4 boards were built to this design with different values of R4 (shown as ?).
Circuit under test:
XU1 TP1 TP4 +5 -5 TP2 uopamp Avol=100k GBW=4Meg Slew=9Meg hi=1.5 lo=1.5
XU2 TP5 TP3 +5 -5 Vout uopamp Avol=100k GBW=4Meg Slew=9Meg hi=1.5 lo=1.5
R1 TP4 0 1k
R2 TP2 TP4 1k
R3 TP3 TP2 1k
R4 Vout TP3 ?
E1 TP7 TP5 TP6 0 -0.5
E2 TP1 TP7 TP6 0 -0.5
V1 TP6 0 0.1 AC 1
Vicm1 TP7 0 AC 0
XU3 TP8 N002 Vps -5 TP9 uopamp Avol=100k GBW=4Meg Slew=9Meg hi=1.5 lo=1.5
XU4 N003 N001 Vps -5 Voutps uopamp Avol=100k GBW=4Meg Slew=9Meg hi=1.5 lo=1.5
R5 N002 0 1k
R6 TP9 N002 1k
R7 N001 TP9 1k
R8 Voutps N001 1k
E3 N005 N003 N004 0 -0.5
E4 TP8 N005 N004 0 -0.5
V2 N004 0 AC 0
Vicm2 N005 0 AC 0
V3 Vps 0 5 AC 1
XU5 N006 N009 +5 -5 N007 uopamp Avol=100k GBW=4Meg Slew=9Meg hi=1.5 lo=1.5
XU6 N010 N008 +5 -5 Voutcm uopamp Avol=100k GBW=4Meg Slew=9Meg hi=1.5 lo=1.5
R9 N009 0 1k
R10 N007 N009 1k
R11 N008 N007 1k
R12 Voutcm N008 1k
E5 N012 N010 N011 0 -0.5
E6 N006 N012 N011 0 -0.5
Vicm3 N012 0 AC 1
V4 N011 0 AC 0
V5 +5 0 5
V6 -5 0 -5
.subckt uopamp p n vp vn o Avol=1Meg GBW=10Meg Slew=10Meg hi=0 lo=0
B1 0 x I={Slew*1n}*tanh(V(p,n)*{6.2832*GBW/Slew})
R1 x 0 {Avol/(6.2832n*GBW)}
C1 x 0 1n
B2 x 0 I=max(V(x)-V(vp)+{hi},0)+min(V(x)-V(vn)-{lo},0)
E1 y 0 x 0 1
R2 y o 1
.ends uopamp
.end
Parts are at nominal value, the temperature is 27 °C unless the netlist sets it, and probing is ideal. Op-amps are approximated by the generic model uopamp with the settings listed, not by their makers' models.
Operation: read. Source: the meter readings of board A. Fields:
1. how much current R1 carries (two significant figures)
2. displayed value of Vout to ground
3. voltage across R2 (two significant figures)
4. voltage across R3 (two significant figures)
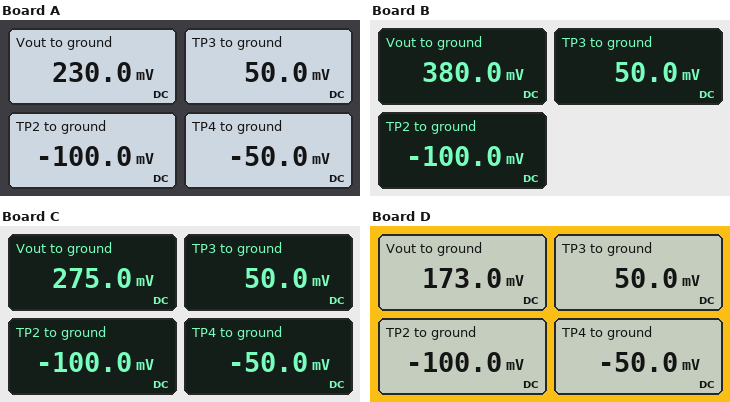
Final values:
50 µA
230.0 mV
50 mV
150 mV
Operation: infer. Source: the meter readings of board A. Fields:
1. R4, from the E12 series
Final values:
1.2 kΩ
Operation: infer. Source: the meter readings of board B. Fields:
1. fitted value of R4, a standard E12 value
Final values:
2.2 kΩ
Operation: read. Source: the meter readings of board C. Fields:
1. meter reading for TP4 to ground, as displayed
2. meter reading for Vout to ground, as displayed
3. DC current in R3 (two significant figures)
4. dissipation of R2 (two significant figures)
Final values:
-50.0 mV
275.0 mV
150 µA
2.5 µW
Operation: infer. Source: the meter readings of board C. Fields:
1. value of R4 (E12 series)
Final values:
1.5 kΩ
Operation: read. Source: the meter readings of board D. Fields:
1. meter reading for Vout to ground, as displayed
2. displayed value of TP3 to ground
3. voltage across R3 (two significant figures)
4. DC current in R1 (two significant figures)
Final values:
173.0 mV
50.0 mV
150 mV
50 µA
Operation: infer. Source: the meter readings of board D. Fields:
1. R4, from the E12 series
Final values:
820 Ω
